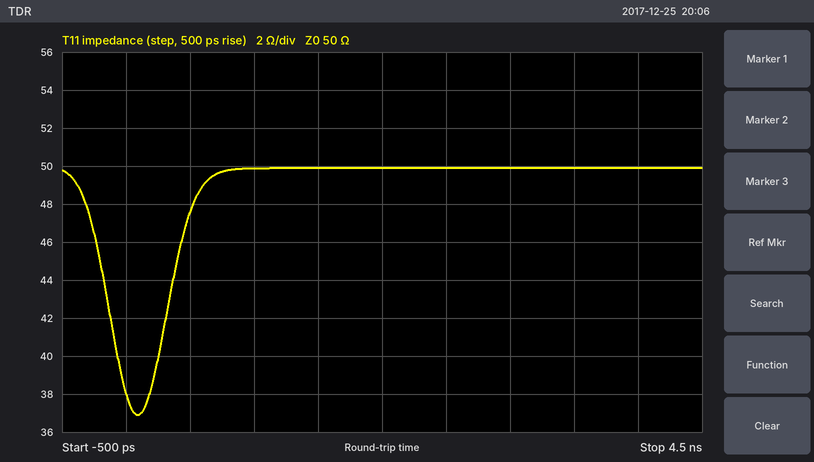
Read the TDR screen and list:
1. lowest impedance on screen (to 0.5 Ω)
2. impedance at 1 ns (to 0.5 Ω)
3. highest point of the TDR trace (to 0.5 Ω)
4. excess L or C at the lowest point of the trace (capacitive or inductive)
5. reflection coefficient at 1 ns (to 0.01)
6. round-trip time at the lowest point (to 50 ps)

37.0 Ω
50.0 Ω
50.0 Ω
capacitive
0.00
100 ps
